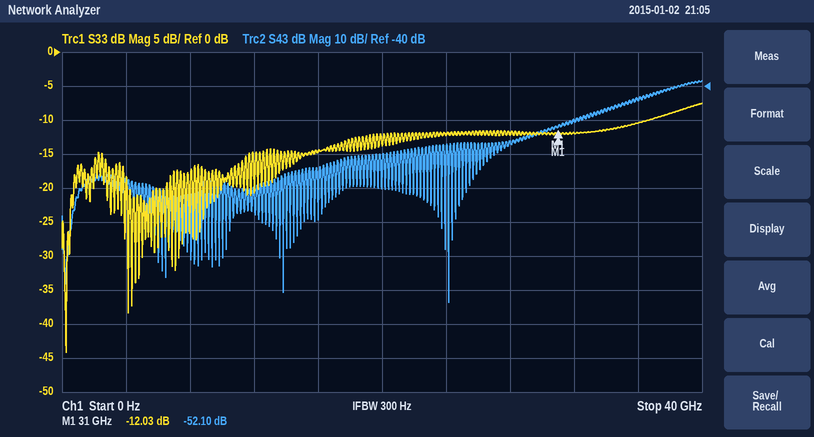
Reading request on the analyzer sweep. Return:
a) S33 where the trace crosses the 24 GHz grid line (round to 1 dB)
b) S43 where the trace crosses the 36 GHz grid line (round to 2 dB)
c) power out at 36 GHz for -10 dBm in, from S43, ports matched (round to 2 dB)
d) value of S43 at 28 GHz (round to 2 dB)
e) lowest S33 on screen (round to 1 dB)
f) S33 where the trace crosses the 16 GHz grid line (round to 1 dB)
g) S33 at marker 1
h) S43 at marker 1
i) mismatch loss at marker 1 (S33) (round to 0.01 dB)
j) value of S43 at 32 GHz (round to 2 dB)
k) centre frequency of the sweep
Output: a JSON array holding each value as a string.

["-12 dB", "-44 dB", "-54 dBm", "-56 dB", "-44 dB", "-15 dB", "-12.03 dB", "-52.10 dB", "0.28 dB", "-50 dB", "20 GHz"]
